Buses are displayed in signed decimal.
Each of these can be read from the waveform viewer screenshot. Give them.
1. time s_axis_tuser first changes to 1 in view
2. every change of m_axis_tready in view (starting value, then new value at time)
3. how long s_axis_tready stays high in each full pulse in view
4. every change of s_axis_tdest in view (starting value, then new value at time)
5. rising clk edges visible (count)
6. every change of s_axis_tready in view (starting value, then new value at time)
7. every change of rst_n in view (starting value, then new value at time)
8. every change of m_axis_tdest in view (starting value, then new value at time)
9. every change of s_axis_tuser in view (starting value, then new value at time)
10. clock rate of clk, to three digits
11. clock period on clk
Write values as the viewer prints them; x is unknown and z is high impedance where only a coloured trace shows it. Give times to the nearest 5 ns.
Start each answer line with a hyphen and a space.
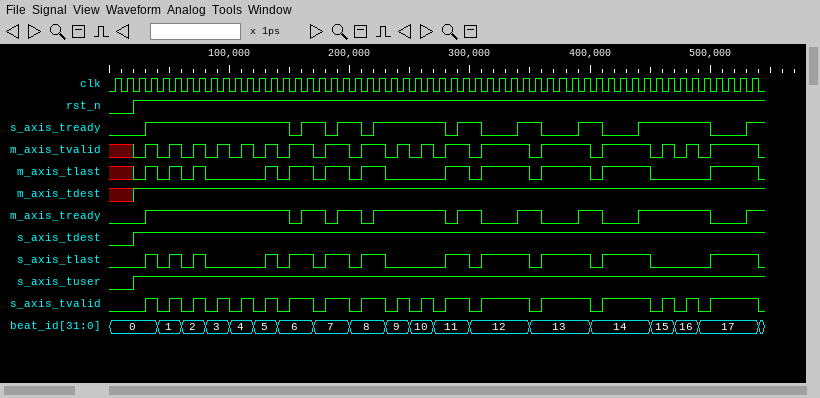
- 20 ns
- 0, 1 at 30 ns, 0 at 150 ns, 1 at 160 ns, 0 at 180 ns, 1 at 190 ns, 0 at 210 ns, 1 at 220 ns, 0 at 280 ns, 1 at 290 ns, 0 at 310 ns, 1 at 340 ns, 0 at 360 ns, 1 at 390 ns, 0 at 410 ns, 1 at 440 ns, 0 at 500 ns, 1 at 530 ns
- 120 ns, 20 ns, 20 ns, 60 ns, 20 ns, 20 ns, 20 ns, 60 ns
- 0, 1 at 20 ns
- 54
- 0, 1 at 30 ns, 0 at 150 ns, 1 at 160 ns, 0 at 180 ns, 1 at 190 ns, 0 at 210 ns, 1 at 220 ns, 0 at 280 ns, 1 at 290 ns, 0 at 310 ns, 1 at 340 ns, 0 at 360 ns, 1 at 390 ns, 0 at 410 ns, 1 at 440 ns, 0 at 500 ns, 1 at 530 ns
- 0, 1 at 20 ns
- x, 1 at 20 ns
- 0, 1 at 20 ns
- 100 MHz
- 10 ns
